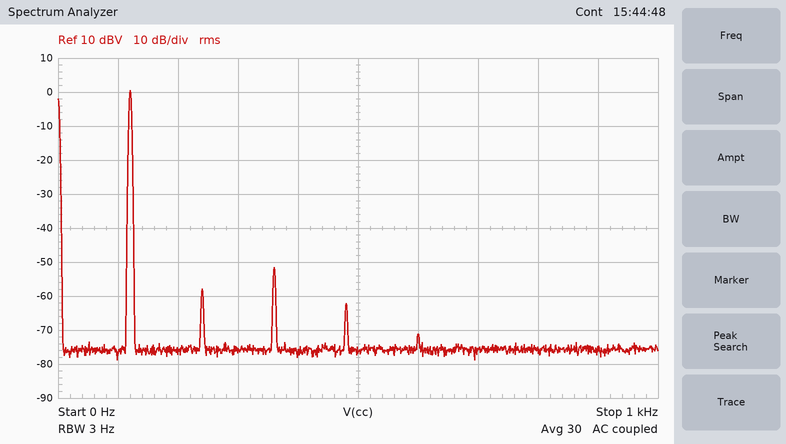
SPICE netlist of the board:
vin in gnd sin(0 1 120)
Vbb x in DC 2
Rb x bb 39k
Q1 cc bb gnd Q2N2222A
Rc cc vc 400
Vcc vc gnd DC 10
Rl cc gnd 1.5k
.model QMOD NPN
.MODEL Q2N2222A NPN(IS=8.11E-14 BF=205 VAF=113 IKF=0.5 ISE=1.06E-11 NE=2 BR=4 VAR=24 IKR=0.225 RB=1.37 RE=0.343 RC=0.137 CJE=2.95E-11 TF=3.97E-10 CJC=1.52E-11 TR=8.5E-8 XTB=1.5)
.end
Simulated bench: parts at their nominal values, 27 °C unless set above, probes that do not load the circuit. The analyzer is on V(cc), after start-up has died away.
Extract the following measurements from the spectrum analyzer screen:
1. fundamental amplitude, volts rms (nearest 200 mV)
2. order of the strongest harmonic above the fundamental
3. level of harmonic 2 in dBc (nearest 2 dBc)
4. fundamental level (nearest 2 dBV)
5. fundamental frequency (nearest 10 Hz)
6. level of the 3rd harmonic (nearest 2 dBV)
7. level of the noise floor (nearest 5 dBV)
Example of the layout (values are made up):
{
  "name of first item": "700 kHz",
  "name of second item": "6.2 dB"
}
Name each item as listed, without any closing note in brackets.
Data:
{
  "fundamental amplitude, volts rms": "1.0 V",
  "order of the strongest harmonic above the fundamental": "3",
  "level of harmonic 2 in dBc": "-58 dBc",
  "fundamental level": "0 dBV",
  "fundamental frequency": "120 Hz",
  "level of the 3rd harmonic": "-52 dBV",
  "level of the noise floor": "-75 dBV"
}
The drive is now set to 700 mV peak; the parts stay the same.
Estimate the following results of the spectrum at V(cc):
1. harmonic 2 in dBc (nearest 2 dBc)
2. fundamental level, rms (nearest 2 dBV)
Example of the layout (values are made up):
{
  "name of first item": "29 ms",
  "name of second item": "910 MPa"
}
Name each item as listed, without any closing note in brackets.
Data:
{
  "harmonic 2 in dBc": "-54 dBc",
  "fundamental level, rms": "-2 dBV"
}
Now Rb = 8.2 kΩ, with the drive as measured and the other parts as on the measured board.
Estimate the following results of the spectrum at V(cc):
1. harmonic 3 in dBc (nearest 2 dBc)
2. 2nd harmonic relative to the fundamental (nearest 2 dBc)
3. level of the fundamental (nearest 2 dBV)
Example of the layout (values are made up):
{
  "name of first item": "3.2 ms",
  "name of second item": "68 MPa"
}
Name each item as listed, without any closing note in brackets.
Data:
{
  "harmonic 3 in dBc": "-20 dBc",
  "2nd harmonic relative to the fundamental": "-6 dBc",
  "level of the fundamental": "4 dBV"
}
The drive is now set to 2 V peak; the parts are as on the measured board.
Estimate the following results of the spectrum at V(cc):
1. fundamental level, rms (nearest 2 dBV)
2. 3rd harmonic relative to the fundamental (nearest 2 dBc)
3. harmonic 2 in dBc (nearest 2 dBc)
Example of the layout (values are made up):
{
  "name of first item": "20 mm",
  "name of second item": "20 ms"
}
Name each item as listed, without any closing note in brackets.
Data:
{
  "fundamental level, rms": "6 dBV",
  "3rd harmonic relative to the fundamental": "-24 dBc",
  "harmonic 2 in dBc": "-22 dBc"
}
